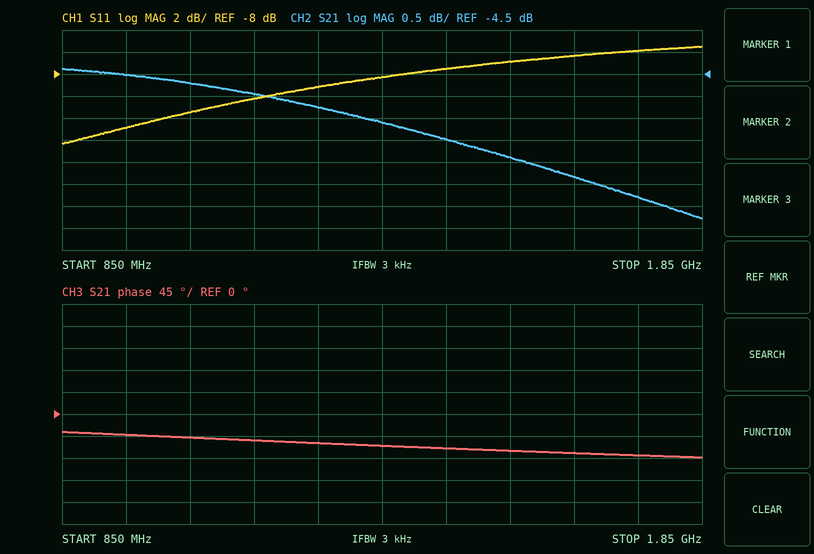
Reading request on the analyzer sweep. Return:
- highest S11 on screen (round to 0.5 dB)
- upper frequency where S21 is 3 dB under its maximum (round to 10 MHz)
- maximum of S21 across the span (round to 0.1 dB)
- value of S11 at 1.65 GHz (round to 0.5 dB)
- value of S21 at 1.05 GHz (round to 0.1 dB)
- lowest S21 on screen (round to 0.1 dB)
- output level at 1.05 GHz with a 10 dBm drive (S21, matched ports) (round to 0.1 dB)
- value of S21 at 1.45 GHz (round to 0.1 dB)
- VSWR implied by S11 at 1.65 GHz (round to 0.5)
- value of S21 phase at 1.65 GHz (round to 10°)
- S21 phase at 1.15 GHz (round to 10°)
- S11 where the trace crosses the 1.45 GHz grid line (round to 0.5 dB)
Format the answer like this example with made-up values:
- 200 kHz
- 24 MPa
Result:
- -5.5 dB
- 1.77 GHz
- -4.4 dB
- -6.5 dB
- -4.7 dB
- -7.8 dB
- 5.3 dBm
- -6.0 dB
- 3.0
- -80°
- -50°
- -7.5 dB
